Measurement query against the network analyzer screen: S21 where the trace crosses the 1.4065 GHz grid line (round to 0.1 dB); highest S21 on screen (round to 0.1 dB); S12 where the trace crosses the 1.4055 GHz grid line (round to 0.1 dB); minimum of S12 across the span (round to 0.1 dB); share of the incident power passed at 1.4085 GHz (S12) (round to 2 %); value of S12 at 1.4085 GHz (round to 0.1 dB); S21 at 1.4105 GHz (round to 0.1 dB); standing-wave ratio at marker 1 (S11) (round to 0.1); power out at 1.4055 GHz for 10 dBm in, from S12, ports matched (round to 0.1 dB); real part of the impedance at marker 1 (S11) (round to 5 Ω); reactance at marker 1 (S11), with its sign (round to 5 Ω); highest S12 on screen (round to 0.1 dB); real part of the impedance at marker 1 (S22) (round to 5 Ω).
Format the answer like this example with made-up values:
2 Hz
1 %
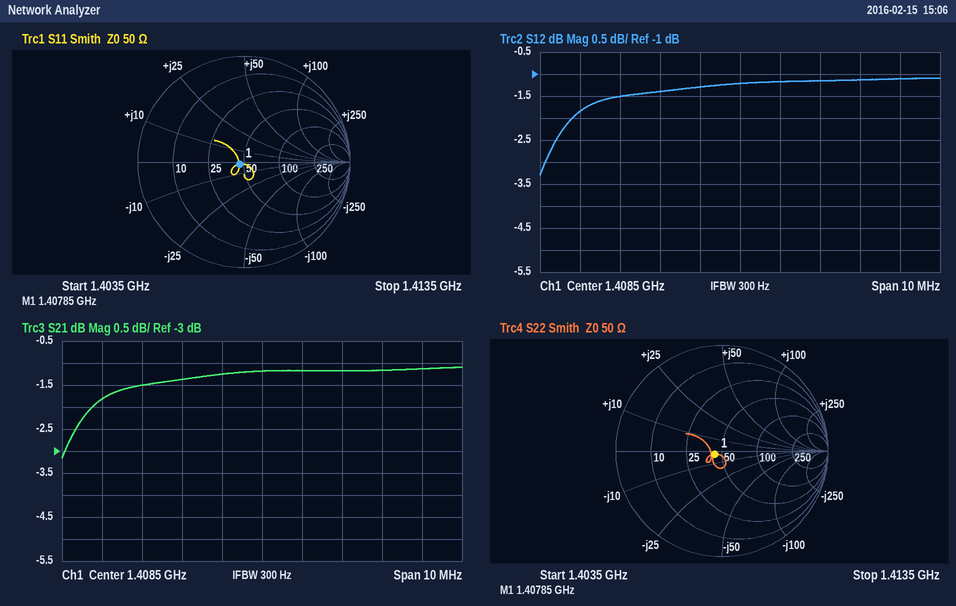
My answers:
-1.4 dB
-1.1 dB
-1.5 dB
-3.3 dB
76 %
-1.2 dB
-1.2 dB
1.1
8.5 dBm
45 Ω
0 Ω
-1.1 dB
45 Ω
